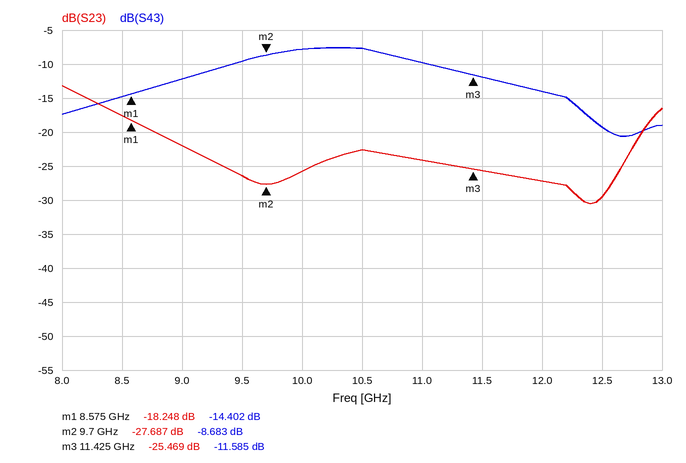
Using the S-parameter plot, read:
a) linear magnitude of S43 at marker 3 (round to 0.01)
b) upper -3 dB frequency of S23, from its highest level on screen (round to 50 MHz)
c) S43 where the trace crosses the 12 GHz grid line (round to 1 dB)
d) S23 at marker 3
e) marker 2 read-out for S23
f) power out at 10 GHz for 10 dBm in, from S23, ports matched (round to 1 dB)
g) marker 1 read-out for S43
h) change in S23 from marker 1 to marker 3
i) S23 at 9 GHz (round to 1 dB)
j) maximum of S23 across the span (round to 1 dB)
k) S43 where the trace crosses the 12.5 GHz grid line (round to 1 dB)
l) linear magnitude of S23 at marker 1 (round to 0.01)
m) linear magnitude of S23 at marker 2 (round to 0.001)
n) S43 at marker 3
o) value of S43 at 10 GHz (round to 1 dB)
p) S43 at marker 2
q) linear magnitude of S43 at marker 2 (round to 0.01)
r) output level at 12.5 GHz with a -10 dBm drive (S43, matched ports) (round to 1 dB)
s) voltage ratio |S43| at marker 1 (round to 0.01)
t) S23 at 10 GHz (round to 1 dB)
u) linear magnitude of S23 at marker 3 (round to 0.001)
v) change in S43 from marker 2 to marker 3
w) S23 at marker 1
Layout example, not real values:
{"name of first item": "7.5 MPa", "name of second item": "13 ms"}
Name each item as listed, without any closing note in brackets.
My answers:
{"linear magnitude of S43 at marker 3": "0.26", "upper -3 dB frequency of S23, from its highest level on screen": "8.35 GHz", "S43 where the trace crosses the 12 GHz grid line": "-14 dB", "S23 at marker 3": "-25.469 dB", "marker 2 read-out for S23": "-27.687 dB", "power out at 10 GHz for 10 dBm in, from S23, ports matched": "-16 dBm", "marker 1 read-out for S43": "-14.402 dB", "change in S23 from marker 1 to marker 3": "-7.221 dB", "S23 at 9 GHz": "-22 dB", "maximum of S23 across the span": "-13 dB", "S43 where the trace crosses the 12.5 GHz grid line": "-19 dB", "linear magnitude of S23 at marker 1": "0.12", "linear magnitude of S23 at marker 2": "0.041", "S43 at marker 3": "-11.585 dB", "value of S43 at 10 GHz": "-8 dB", "S43 at marker 2": "-8.683 dB", "linear magnitude of S43 at marker 2": "0.37", "output level at 12.5 GHz with a -10 dBm drive (S43, matched ports)": "-29 dBm", "voltage ratio |S43| at marker 1": "0.19", "S23 at 10 GHz": "-26 dB", "linear magnitude of S23 at marker 3": "0.053", "change in S43 from marker 2 to marker 3": "-2.902 dB", "S23 at marker 1": "-18.248 dB"}
